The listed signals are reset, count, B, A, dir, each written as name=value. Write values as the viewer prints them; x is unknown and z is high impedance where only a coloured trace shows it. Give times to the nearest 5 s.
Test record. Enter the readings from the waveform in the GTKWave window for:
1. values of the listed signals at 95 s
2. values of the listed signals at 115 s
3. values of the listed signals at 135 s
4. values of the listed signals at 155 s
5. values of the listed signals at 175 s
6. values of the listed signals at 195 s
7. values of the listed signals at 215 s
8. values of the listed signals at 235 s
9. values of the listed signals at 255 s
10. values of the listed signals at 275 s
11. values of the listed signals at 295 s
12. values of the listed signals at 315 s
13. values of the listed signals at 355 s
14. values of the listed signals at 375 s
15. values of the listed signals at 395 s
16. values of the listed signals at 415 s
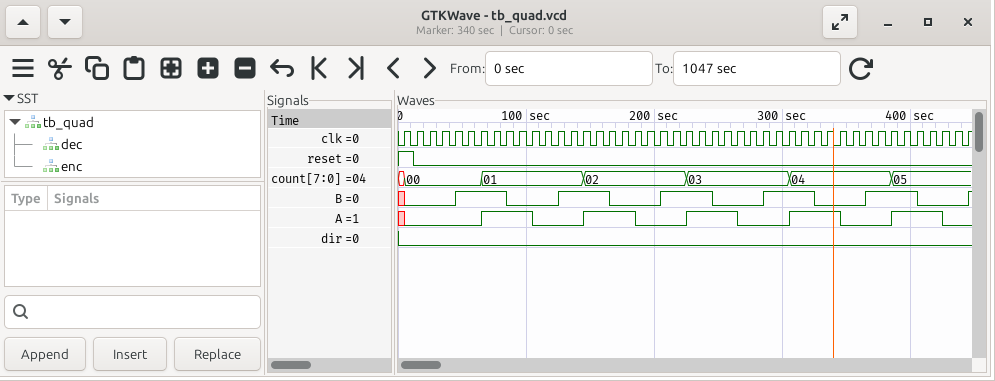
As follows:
reset=0, count=01, B=0, A=1, dir=0
reset=0, count=01, B=0, A=0, dir=0
reset=0, count=01, B=1, A=0, dir=0
reset=0, count=02, B=1, A=1, dir=0
reset=0, count=02, B=0, A=1, dir=0
reset=0, count=02, B=0, A=0, dir=0
reset=0, count=02, B=1, A=0, dir=0
reset=0, count=03, B=1, A=1, dir=0
reset=0, count=03, B=0, A=1, dir=0
reset=0, count=03, B=0, A=0, dir=0
reset=0, count=03, B=1, A=0, dir=0
reset=0, count=04, B=1, A=1, dir=0
reset=0, count=04, B=0, A=0, dir=0
reset=0, count=04, B=1, A=0, dir=0
reset=0, count=05, B=1, A=1, dir=0
reset=0, count=05, B=0, A=1, dir=0
